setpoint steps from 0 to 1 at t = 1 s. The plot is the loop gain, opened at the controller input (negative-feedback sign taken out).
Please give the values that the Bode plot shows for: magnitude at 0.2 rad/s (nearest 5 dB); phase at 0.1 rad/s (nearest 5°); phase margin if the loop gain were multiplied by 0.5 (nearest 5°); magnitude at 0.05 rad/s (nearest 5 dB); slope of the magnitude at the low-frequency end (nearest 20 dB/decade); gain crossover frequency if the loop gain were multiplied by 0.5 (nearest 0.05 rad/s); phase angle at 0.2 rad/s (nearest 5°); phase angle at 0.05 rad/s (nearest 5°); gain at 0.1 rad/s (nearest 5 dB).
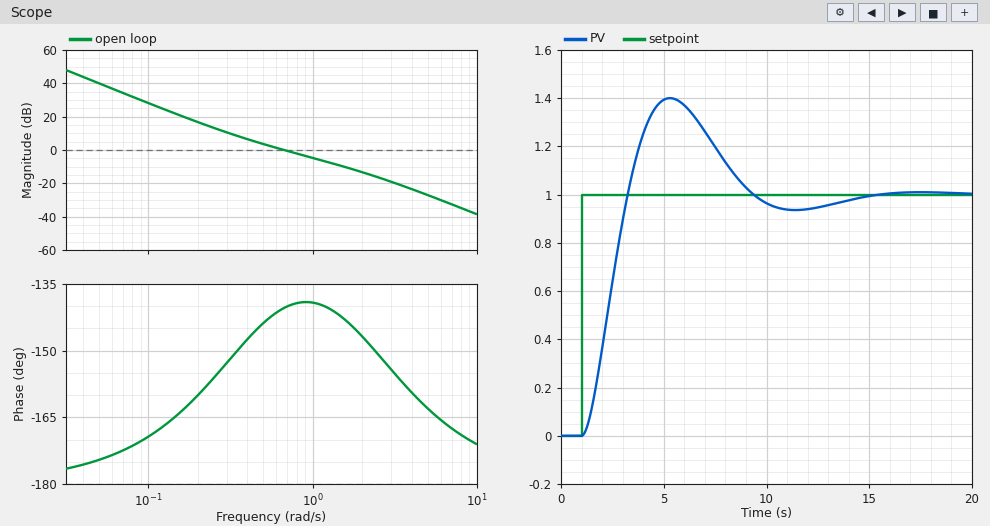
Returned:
15 dB
-170°
35°
40 dB
-40 dB/decade
0.40 rad/s
-160°
-175°
30 dB
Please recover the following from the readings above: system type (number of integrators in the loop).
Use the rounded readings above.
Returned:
2
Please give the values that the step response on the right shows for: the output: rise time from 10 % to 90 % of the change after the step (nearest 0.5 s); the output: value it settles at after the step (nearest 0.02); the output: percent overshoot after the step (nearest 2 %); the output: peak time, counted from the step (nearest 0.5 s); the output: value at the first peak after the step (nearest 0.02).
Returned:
1.5 s
1.00
40 %
4.5 s
1.40
